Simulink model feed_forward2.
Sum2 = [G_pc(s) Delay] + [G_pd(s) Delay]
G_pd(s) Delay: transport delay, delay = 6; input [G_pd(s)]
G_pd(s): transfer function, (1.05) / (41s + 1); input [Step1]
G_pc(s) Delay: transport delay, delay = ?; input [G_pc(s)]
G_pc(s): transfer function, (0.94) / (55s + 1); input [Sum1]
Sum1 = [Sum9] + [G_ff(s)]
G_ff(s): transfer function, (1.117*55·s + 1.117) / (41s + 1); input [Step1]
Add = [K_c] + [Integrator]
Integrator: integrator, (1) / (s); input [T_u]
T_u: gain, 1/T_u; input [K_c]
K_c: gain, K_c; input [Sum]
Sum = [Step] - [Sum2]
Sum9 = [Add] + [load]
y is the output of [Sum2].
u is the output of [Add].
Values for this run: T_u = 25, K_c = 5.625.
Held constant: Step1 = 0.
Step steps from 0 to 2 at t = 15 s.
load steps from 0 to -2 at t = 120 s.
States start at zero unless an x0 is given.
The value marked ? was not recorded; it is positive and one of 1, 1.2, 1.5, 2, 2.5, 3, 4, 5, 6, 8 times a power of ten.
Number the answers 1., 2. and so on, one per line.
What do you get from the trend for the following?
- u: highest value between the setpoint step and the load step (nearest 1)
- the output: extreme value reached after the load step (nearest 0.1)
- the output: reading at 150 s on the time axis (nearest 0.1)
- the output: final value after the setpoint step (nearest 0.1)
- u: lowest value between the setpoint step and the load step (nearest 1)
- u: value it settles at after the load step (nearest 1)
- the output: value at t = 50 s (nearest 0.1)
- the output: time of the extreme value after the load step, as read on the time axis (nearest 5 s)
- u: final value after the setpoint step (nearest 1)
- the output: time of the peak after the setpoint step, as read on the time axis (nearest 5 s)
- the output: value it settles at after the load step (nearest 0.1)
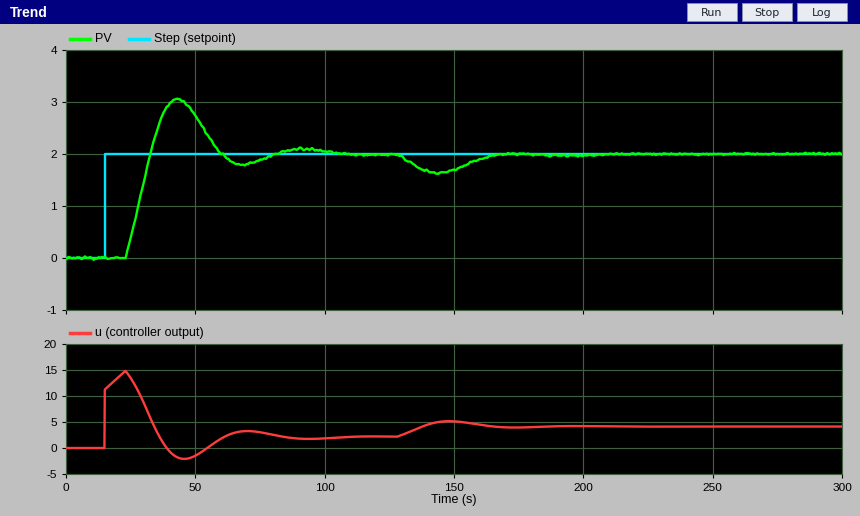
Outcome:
1. 15
2. 1.6
3. 1.7
4. 2.0
5. -2
6. 4
7. 2.7
8. 145 s
9. 2
10. 45 s
11. 2.0
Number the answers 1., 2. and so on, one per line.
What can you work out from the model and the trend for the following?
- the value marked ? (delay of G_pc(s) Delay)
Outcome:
1. 8
